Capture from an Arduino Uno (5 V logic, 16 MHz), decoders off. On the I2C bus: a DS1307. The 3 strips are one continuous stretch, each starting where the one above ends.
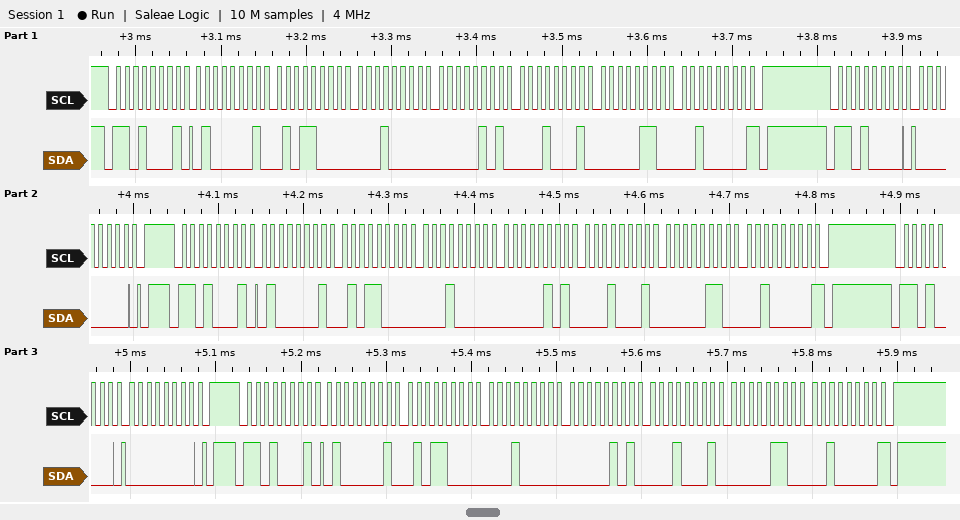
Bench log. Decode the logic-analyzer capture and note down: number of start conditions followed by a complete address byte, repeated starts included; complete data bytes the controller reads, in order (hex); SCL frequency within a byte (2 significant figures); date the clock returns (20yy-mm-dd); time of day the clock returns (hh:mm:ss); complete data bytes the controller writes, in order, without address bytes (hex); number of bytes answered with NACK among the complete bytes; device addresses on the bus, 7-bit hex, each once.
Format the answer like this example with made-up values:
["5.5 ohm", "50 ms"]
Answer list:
["5", "41 58 10 05 11 06 20 41 58 10 05 11 06 20 41 58 10 05 11 06 20", "100 kHz", "2020-06-11", "10:58:41", "00 00", "3", "0x68"]
